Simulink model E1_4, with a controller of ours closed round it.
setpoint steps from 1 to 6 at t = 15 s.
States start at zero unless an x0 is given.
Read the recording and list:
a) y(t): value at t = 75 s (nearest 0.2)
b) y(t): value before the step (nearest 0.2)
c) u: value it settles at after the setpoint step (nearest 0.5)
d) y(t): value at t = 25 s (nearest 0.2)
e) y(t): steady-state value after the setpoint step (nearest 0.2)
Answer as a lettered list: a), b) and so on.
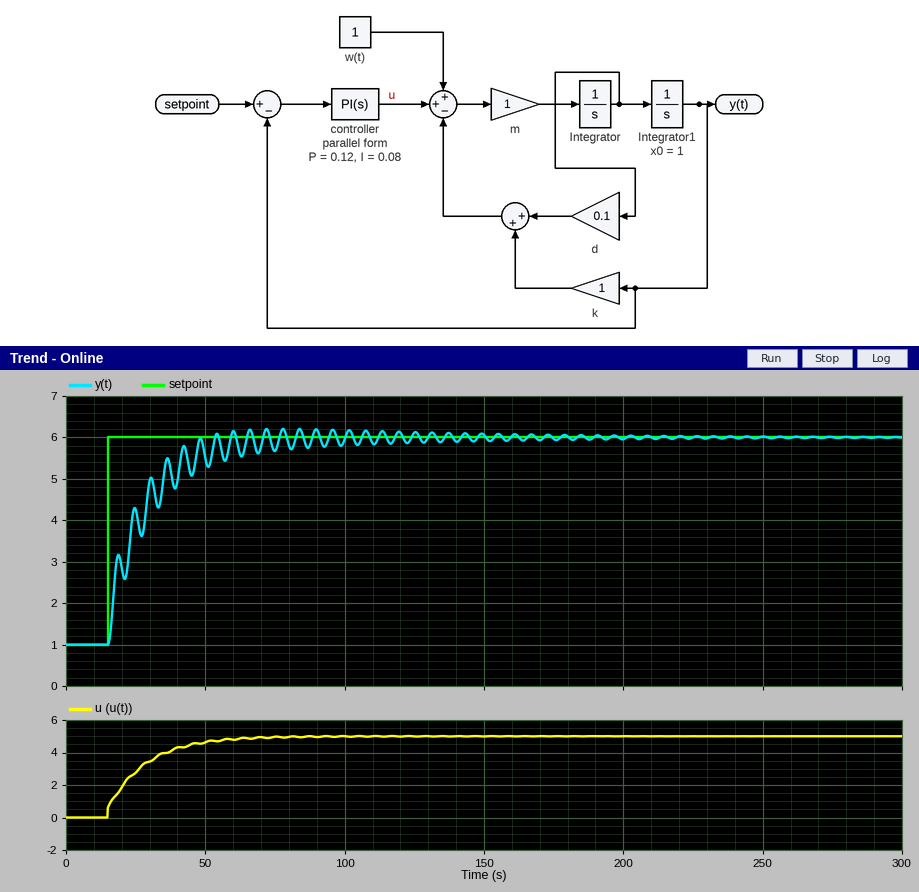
a) 5.6
b) 1.0
c) 5.0
d) 4.2
e) 6.0
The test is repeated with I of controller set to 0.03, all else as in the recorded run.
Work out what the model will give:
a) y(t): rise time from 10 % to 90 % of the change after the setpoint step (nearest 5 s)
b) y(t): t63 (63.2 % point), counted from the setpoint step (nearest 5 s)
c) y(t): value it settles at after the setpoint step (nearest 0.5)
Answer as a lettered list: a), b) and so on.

a) 80 s
b) 30 s
c) 6.0
